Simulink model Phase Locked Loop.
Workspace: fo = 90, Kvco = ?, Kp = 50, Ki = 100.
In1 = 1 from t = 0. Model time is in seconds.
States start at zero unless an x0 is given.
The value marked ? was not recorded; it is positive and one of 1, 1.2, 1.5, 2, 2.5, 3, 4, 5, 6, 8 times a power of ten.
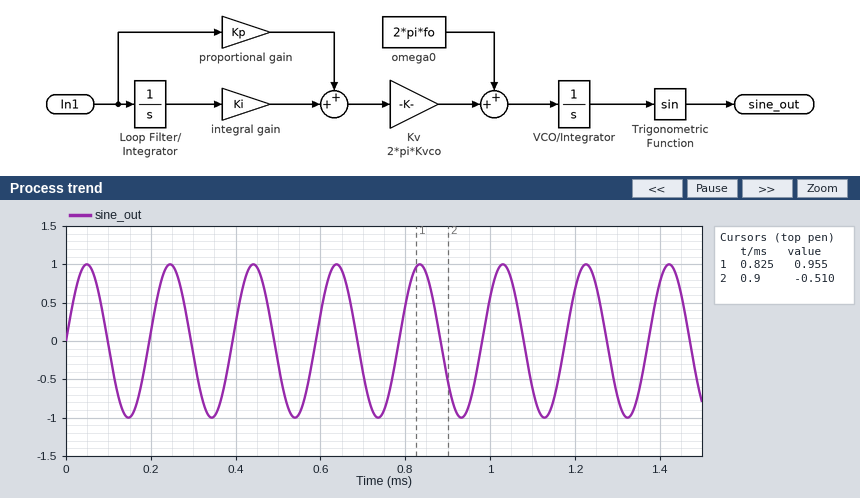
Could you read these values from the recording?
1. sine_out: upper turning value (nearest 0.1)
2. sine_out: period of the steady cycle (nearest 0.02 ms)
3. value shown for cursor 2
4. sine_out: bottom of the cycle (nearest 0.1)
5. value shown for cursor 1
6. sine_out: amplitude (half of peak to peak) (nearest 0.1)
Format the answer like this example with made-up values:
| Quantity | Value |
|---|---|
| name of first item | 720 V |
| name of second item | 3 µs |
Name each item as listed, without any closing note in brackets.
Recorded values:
| Quantity | Value |
|---|---|
| sine_out: upper turning value | 1.0 |
| sine_out: period of the steady cycle | 0.20 ms |
| value shown for cursor 2 | -0.510 |
| sine_out: bottom of the cycle | -1.0 |
| value shown for cursor 1 | 0.955 |
| sine_out: amplitude (half of peak to peak) | 1.0 |
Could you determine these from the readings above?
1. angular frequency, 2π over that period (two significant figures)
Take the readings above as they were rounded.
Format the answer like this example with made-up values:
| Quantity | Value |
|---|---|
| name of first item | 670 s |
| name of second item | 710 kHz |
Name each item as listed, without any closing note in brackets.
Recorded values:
| Quantity | Value |
|---|---|
| angular frequency, 2π over that period | 31 rad/ms |
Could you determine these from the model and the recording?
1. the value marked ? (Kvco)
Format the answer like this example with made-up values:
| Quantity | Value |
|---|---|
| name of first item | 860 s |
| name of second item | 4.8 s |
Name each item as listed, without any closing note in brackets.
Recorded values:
| Quantity | Value |
|---|---|
| the value marked ? | 100 |
